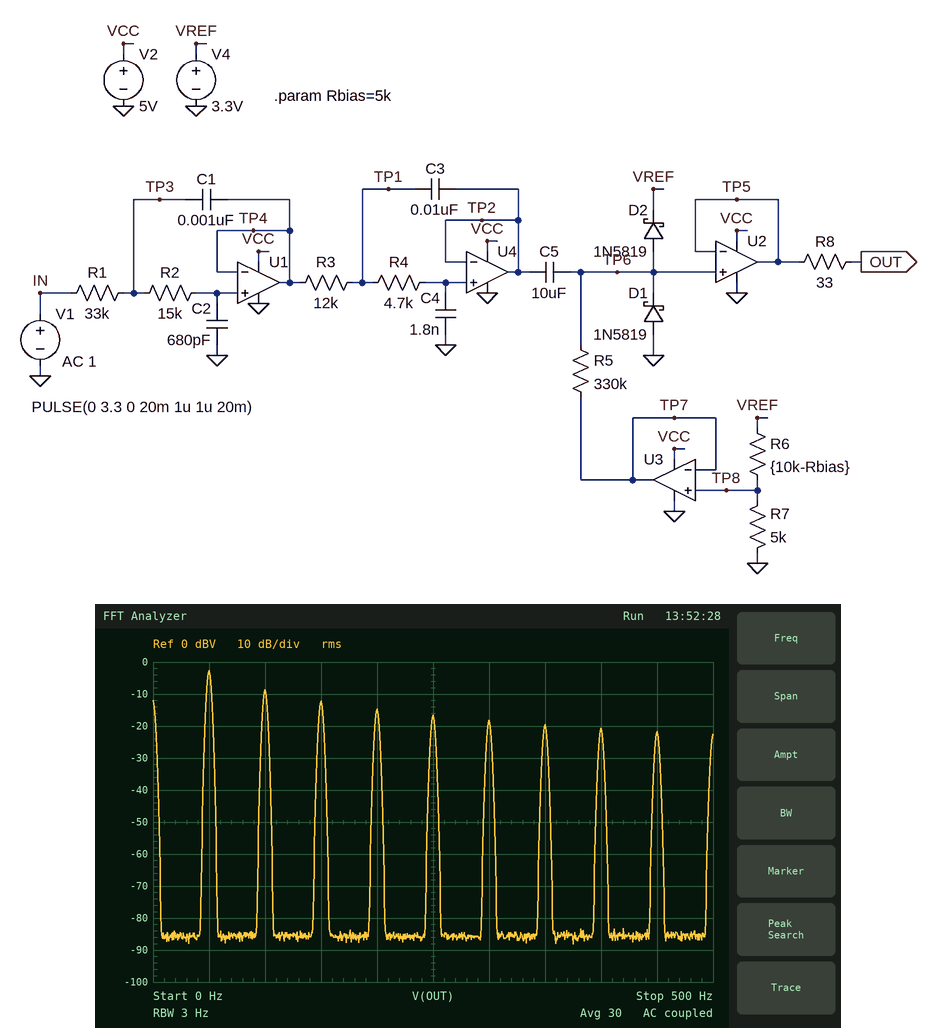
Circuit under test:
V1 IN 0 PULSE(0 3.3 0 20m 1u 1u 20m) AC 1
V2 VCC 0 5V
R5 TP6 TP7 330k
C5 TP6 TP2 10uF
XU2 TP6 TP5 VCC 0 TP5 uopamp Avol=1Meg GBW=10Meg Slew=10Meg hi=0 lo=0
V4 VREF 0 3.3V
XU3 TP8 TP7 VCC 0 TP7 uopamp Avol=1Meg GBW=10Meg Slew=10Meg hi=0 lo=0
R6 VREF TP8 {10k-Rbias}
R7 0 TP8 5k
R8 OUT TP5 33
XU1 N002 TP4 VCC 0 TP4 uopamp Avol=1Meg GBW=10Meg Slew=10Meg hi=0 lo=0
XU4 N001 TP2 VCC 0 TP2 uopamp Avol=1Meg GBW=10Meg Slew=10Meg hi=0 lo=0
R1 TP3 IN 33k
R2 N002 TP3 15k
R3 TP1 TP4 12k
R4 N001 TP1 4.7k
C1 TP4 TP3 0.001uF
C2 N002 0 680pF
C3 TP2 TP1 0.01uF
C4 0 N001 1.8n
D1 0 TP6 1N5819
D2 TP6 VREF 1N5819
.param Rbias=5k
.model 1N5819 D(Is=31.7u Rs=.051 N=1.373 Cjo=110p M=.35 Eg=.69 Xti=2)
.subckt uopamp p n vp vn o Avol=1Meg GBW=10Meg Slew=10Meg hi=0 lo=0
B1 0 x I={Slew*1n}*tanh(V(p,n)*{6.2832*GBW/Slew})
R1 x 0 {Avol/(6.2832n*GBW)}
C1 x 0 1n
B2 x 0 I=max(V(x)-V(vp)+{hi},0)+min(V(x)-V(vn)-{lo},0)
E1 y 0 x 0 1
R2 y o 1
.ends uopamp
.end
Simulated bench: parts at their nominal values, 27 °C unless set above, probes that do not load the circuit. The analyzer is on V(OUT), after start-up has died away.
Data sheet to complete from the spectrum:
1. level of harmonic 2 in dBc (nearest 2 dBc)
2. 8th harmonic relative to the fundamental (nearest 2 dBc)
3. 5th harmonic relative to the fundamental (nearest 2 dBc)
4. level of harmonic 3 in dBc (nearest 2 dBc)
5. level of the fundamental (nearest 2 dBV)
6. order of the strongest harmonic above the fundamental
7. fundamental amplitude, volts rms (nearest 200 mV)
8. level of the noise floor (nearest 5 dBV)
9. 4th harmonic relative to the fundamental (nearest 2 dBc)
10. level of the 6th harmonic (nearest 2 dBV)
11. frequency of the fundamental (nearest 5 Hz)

-6 dBc
-18 dBc
-14 dBc
-10 dBc
-2 dBV
2
800 mV
-85 dBV
-12 dBc
-18 dBV
50 Hz
